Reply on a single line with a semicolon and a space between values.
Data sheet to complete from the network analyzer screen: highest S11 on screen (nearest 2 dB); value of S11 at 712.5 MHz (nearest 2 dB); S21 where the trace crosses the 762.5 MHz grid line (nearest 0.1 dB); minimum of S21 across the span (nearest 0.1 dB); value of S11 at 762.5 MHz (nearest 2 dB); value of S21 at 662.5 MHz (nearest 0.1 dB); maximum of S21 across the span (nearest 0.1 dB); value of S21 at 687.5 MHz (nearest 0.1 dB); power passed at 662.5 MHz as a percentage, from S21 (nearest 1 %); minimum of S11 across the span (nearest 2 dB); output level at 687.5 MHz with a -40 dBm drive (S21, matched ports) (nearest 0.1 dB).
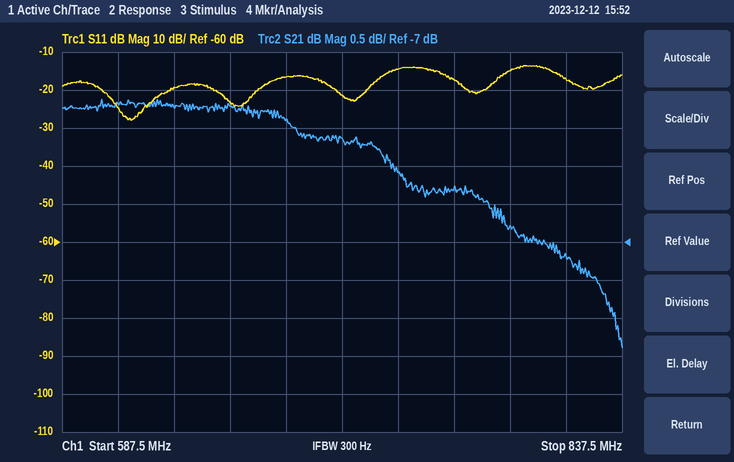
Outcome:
-14 dB; -22 dB; -6.3 dB; -8.4 dB; -18 dB; -5.2 dB; -5.1 dB; -5.4 dB; 30 %; -28 dB; -45.4 dBm
